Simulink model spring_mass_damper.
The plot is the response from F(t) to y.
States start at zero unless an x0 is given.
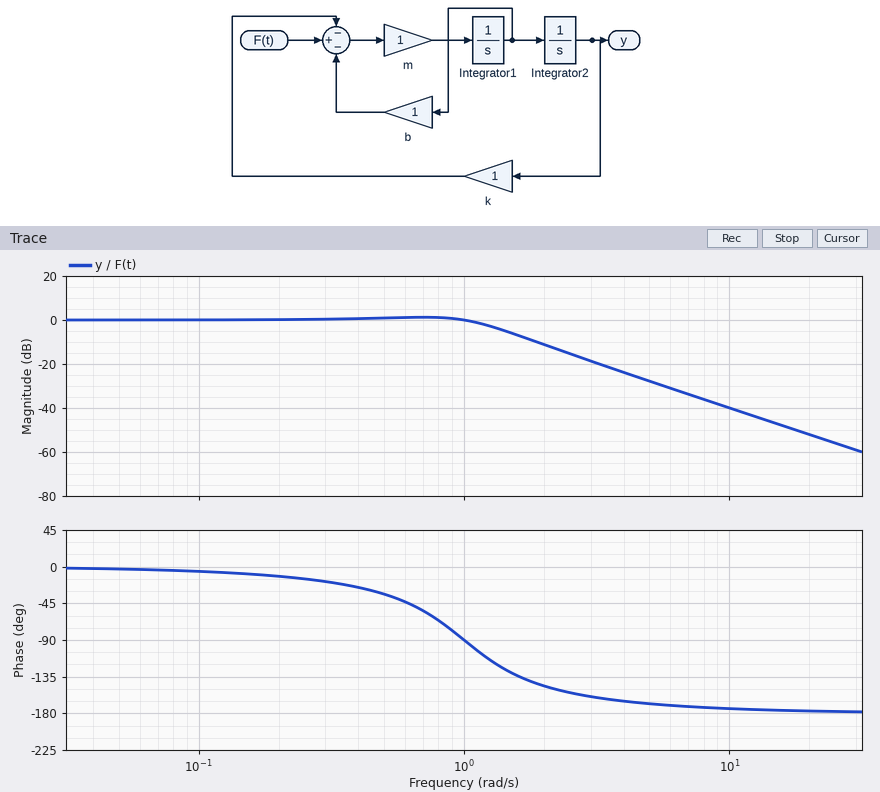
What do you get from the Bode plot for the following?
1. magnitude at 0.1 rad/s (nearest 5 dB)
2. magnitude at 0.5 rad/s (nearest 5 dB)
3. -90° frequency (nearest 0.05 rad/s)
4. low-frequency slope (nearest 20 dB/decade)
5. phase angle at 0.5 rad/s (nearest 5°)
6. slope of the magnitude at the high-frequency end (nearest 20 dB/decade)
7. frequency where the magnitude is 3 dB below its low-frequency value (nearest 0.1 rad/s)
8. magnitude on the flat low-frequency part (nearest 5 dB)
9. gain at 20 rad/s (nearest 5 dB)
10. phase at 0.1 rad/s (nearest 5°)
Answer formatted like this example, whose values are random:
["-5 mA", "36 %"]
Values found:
["0 dB", "0 dB", "1.00 rad/s", "0 dB/decade", "-35°", "-40 dB/decade", "1.3 rad/s", "0 dB", "-50 dB", "-5°"]
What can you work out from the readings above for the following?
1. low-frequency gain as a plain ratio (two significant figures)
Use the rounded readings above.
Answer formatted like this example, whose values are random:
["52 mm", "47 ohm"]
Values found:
["1.0"]
